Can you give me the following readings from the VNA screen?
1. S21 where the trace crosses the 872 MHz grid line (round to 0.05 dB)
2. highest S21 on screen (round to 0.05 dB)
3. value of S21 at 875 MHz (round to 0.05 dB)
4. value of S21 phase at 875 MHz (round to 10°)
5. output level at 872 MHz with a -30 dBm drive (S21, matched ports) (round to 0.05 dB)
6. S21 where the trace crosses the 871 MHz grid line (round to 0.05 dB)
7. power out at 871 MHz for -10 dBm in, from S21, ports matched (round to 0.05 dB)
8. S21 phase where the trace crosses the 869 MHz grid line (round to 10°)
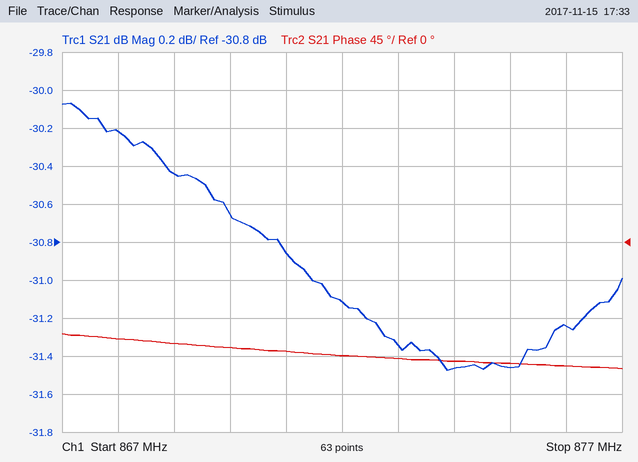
-31.10 dB
-30.05 dB
-31.45 dB
-140°
-61.10 dBm
-30.85 dB
-40.85 dBm
-120°
